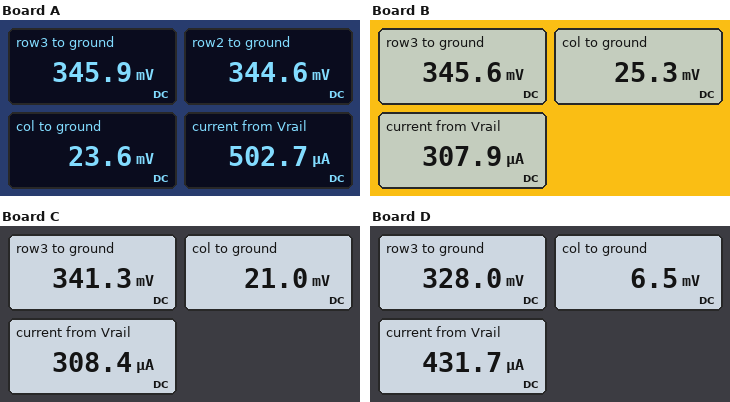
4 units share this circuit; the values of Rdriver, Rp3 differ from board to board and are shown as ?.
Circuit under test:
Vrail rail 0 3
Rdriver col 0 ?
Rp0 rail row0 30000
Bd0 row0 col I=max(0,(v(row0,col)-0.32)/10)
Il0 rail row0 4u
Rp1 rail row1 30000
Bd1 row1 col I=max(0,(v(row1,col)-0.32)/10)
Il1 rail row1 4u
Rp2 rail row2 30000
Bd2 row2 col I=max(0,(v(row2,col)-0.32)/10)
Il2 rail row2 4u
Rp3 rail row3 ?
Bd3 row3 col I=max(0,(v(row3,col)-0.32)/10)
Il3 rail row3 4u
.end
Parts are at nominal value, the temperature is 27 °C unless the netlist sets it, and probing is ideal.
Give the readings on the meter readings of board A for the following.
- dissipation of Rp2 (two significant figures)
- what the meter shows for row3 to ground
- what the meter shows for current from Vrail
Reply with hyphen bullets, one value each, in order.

- 240 µW
- 345.9 mV
- 502.7 µA
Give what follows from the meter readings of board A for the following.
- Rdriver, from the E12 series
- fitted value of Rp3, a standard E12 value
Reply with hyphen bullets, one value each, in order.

- 47 Ω
- 12 kΩ
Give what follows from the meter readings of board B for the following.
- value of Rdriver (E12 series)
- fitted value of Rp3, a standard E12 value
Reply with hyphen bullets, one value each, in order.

- 82 Ω
- 100 kΩ
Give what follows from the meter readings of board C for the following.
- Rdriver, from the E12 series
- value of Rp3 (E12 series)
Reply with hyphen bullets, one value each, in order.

- 68 Ω
- 100 kΩ
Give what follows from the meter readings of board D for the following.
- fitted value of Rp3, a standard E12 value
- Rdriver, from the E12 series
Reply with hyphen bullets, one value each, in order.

- 18 kΩ
- 15 Ω
